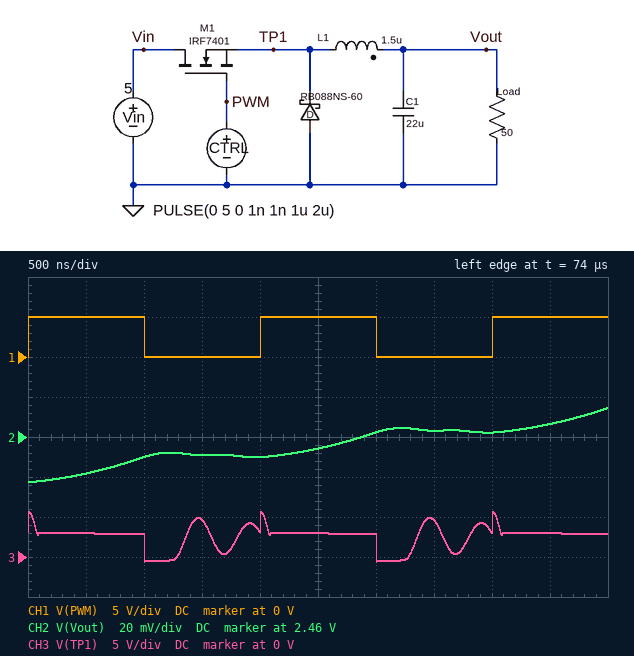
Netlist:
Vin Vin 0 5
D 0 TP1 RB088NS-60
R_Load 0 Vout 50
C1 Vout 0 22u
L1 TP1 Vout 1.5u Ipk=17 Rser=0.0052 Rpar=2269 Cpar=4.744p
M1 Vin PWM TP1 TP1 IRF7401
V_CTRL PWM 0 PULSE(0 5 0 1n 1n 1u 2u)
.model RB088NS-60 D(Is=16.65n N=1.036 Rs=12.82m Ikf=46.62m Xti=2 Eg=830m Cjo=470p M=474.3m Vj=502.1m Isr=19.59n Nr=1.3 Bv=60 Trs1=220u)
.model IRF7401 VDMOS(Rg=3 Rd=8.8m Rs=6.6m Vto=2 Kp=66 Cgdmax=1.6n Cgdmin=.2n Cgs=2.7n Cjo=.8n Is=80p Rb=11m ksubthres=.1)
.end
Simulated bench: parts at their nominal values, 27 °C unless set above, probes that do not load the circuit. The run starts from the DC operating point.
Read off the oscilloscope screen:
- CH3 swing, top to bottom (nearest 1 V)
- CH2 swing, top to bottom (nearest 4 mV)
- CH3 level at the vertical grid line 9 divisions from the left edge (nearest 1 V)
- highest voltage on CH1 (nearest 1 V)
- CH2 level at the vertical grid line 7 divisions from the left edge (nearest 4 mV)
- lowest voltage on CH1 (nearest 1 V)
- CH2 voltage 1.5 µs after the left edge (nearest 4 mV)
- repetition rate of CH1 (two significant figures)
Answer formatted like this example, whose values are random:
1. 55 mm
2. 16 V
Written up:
1. 6 V
2. 36 mV
3. 3 V
4. 5 V
5. 2.464 V
6. 0 V
7. 2.452 V
8. 500 kHz
